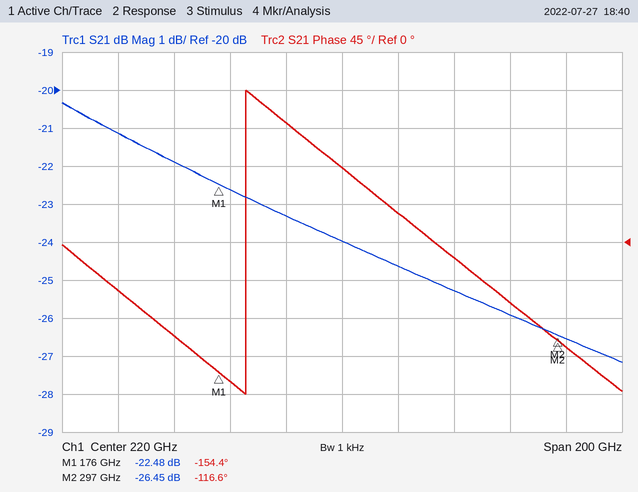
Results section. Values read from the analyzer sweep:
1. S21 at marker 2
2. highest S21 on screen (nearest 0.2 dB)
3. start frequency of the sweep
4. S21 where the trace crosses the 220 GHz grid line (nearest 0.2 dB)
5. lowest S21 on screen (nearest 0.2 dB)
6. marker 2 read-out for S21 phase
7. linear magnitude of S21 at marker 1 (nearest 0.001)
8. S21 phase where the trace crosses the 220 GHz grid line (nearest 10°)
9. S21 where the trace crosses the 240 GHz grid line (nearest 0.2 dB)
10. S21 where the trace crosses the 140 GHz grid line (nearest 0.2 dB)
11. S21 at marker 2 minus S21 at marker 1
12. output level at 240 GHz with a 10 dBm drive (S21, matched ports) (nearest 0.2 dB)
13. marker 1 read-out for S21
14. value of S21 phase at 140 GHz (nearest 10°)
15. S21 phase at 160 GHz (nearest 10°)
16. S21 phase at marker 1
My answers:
-26.45 dB
-20.4 dB
120 GHz
-24.0 dB
-27.2 dB
-116.6°
0.075
90°
-24.6 dB
-21.2 dB
-3.97 dB
-14.6 dBm
-22.48 dB
-60°
-110°
-154.4°
